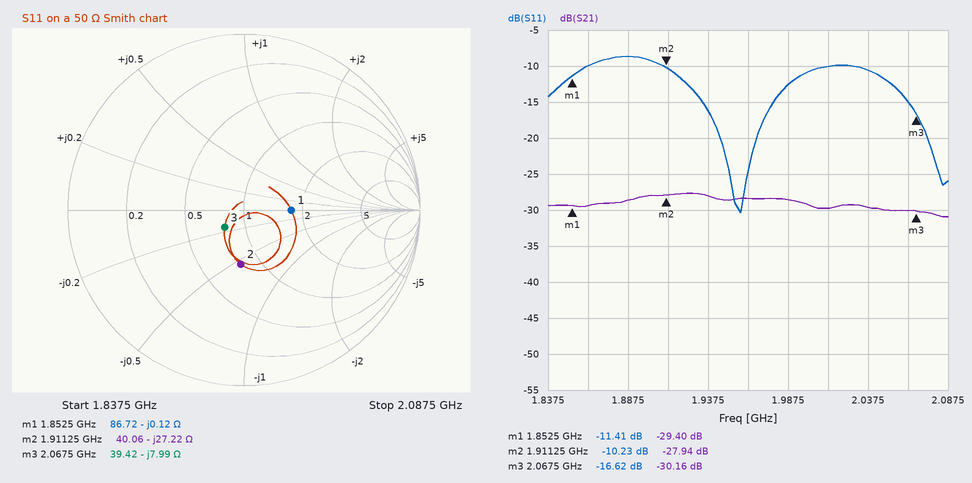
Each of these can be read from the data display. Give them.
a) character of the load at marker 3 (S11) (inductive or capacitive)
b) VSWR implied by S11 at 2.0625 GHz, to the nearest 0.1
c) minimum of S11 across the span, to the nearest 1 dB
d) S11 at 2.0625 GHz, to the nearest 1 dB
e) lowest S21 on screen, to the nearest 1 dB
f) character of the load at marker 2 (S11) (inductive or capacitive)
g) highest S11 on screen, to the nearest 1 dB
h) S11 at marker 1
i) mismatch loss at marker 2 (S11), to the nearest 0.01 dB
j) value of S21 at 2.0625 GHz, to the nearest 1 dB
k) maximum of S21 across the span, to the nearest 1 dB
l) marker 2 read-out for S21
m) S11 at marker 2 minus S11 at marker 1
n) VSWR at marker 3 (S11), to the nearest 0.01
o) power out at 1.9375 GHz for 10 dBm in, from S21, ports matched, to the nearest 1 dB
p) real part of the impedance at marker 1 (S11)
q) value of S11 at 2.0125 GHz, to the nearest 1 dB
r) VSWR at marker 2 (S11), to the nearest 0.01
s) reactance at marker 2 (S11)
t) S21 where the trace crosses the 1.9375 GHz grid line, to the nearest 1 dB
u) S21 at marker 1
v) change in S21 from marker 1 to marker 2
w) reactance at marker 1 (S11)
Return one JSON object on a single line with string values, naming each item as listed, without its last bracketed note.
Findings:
{"character of the load at marker 3 (S11)": "capacitive", "VSWR implied by S11 at 2.0625 GHz, to the nearest 0.1": "1.4", "minimum of S11 across the span, to the nearest 1 dB": "-30 dB", "S11 at 2.0625 GHz, to the nearest 1 dB": "-15 dB", "lowest S21 on screen, to the nearest 1 dB": "-31 dB", "character of the load at marker 2 (S11)": "capacitive", "highest S11 on screen, to the nearest 1 dB": "-9 dB", "S11 at marker 1": "-11.41 dB", "mismatch loss at marker 2 (S11), to the nearest 0.01 dB": "0.43 dB", "value of S21 at 2.0625 GHz, to the nearest 1 dB": "-30 dB", "maximum of S21 across the span, to the nearest 1 dB": "-28 dB", "marker 2 read-out for S21": "-27.94 dB", "S11 at marker 2 minus S11 at marker 1": "1.18 dB", "VSWR at marker 3 (S11), to the nearest 0.01": "1.35", "power out at 1.9375 GHz for 10 dBm in, from S21, ports matched, to the nearest 1 dB": "-18 dBm", "real part of the impedance at marker 1": "86.72 Ω", "value of S11 at 2.0125 GHz, to the nearest 1 dB": "-10 dB", "VSWR at marker 2 (S11), to the nearest 0.01": "1.89", "reactance at marker 2": "-27.22 Ω", "S21 where the trace crosses the 1.9375 GHz grid line, to the nearest 1 dB": "-28 dB", "S21 at marker 1": "-29.40 dB", "change in S21 from marker 1 to marker 2": "1.46 dB", "reactance at marker 1": "-0.12 Ω"}
